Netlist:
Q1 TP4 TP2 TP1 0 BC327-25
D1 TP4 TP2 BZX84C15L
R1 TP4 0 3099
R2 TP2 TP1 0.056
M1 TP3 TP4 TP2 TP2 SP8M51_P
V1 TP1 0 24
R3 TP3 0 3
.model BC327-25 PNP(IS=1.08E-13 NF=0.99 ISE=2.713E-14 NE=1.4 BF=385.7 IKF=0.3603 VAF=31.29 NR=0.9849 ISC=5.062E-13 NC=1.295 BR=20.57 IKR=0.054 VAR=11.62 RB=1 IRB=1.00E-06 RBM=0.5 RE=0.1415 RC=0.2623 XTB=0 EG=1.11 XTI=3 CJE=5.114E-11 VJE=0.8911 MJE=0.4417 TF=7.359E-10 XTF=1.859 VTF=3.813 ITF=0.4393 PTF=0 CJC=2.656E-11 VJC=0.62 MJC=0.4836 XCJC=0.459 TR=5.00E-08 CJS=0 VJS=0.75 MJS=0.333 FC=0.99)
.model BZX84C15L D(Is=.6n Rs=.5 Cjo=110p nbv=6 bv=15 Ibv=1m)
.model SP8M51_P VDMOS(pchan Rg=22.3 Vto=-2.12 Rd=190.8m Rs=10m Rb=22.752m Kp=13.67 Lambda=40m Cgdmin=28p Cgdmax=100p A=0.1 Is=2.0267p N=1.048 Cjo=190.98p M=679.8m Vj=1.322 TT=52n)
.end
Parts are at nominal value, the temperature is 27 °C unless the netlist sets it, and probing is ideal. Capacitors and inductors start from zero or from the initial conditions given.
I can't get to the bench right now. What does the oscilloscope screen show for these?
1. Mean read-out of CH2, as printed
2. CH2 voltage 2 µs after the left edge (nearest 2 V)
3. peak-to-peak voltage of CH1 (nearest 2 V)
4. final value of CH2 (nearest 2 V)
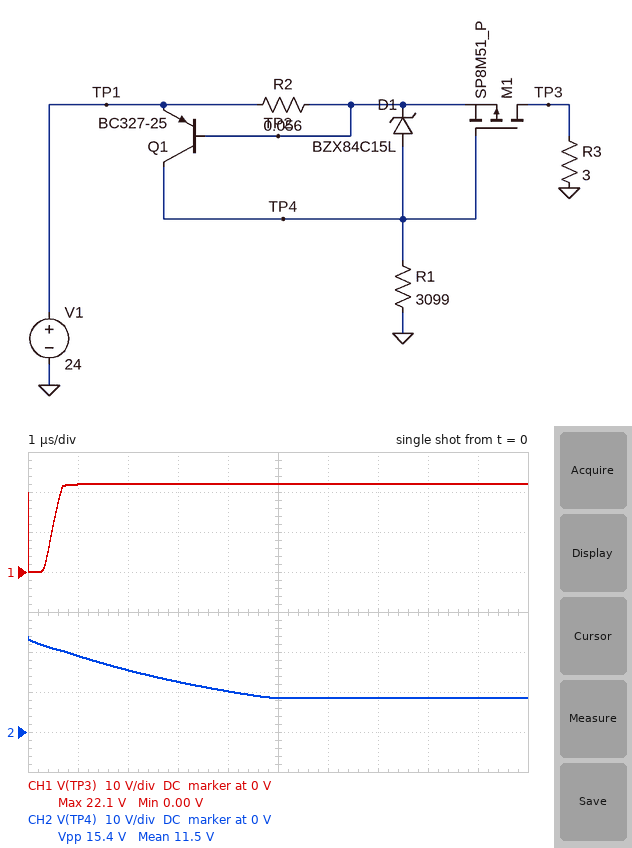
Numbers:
11.5 V
16 V
22 V
8 V
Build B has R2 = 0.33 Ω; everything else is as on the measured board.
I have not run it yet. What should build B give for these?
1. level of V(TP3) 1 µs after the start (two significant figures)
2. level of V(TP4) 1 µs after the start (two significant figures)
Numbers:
5.8 V
21 V
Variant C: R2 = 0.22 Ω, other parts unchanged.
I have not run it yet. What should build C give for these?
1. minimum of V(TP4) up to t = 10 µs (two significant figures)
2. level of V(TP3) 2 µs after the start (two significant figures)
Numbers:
21 V
8.7 V
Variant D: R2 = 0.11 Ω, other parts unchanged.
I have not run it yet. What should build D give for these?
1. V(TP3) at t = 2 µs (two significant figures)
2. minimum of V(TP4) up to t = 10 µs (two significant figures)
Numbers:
17 V
20 V
